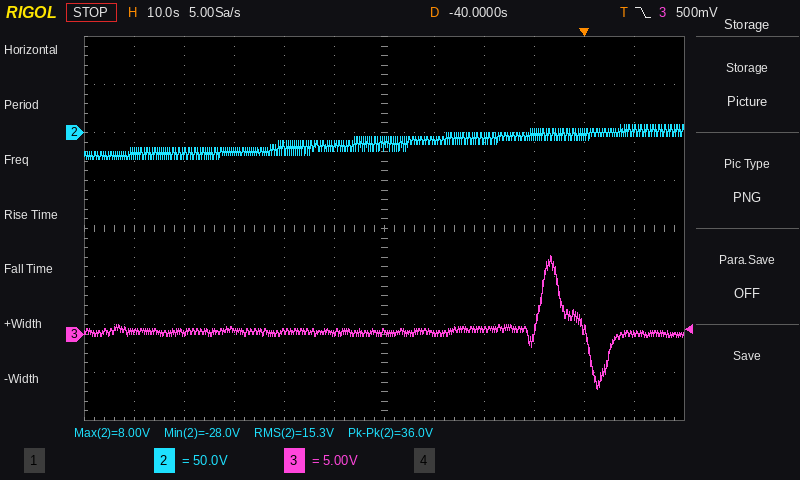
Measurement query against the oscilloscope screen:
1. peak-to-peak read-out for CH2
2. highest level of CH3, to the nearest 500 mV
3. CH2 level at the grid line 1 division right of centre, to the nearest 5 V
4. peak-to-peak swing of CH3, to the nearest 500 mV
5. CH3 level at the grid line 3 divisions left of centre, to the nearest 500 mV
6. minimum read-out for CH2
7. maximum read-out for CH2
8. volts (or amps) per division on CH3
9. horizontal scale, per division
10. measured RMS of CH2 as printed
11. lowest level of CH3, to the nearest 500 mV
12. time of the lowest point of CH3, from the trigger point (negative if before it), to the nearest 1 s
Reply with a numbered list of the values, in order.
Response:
1. 36.0 V
2. 8.0 V
3. -10 V
4. 14.0 V
5. 500 mV
6. -28.0 V
7. 8.00 V
8. 5 V
9. 10 s
10. 15.3 V
11. -6.0 V
12. +3 s
